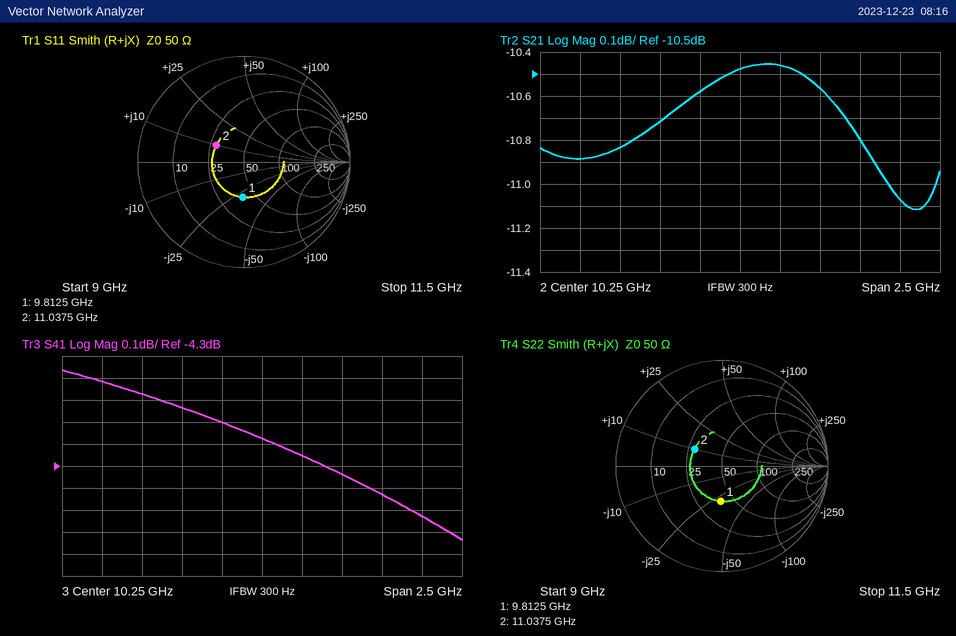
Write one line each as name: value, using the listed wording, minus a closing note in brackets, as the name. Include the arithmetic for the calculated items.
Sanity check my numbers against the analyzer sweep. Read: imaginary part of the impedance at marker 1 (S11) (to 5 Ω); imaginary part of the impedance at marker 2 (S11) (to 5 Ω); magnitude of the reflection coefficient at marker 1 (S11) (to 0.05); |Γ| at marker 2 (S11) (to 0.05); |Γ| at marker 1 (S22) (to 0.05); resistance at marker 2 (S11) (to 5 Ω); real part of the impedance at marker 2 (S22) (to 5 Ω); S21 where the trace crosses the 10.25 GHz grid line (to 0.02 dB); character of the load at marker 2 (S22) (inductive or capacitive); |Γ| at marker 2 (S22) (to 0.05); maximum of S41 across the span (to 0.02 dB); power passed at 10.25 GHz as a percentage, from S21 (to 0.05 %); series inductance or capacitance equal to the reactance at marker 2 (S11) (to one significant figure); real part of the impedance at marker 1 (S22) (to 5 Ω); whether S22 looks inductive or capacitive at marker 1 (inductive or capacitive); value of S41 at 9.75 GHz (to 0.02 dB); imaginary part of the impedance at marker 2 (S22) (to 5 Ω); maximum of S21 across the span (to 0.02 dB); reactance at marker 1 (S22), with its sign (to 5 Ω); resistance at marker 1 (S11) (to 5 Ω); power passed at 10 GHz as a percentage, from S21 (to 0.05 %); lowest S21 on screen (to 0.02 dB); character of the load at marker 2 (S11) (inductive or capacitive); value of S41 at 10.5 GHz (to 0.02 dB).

imaginary part of the impedance at marker 1 (S11): -30 Ω
imaginary part of the impedance at marker 2 (S11): +10 Ω
magnitude of the reflection coefficient at marker 1 (S11): 0.35
|Γ| at marker 2 (S11): 0.30
|Γ| at marker 1 (S22): 0.35
resistance at marker 2 (S11): 30 Ω
real part of the impedance at marker 2 (S22): 30 Ω
S21 where the trace crosses the 10.25 GHz grid line: -10.48 dB
character of the load at marker 2 (S22): inductive
|Γ| at marker 2 (S22): 0.30
maximum of S41 across the span: -3.86 dB
power passed at 10.25 GHz as a percentage, from S21: 10^(-10.48/10) ≈ 8.95 %
series inductance or capacitance equal to the reactance at marker 2 (S11): L = 10 Ω/(2π × 11.0375 GHz) ≈ 144 pH, so 100 pH to one significant figure
real part of the impedance at marker 1 (S22): 40 Ω
whether S22 looks inductive or capacitive at marker 1: capacitive
value of S41 at 9.75 GHz: -4.04 dB
imaginary part of the impedance at marker 2 (S22): +10 Ω
maximum of S21 across the span: -10.46 dB
reactance at marker 1 (S22), with its sign: -30 Ω
resistance at marker 1 (S11): 40 Ω
power passed at 10 GHz as a percentage, from S21: 10^(-10.58/10) ≈ 8.75 %
lowest S21 on screen: -11.12 dB
character of the load at marker 2 (S11): inductive
value of S41 at 10.5 GHz: -4.26 dB
